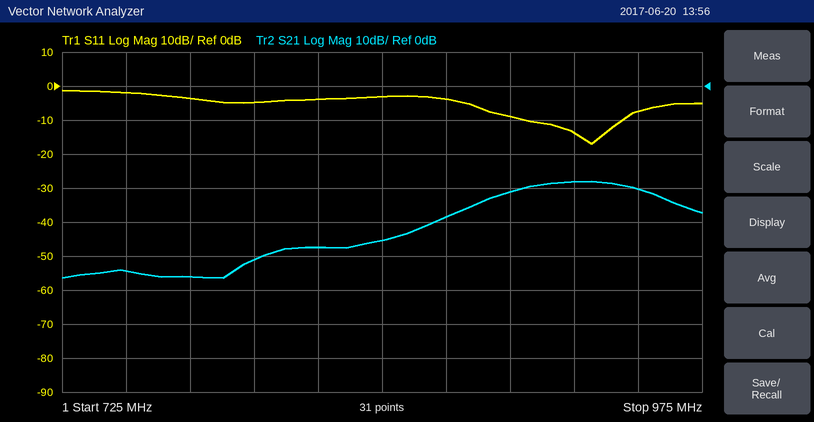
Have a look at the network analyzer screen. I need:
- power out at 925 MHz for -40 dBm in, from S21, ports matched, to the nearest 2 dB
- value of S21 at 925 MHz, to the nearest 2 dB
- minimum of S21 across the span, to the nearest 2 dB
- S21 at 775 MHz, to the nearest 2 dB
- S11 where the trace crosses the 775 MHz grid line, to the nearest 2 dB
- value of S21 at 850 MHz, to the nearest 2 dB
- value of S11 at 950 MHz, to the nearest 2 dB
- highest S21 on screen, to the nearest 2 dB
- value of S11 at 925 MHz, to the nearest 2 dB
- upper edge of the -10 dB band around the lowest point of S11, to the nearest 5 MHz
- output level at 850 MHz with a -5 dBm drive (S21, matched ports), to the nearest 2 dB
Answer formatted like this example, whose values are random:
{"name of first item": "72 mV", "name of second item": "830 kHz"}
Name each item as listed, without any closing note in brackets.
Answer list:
{"power out at 925 MHz for -40 dBm in, from S21, ports matched, to the nearest 2 dB": "-68 dBm", "value of S21 at 925 MHz, to the nearest 2 dB": "-28 dB", "minimum of S21 across the span, to the nearest 2 dB": "-56 dB", "S21 at 775 MHz, to the nearest 2 dB": "-56 dB", "S11 where the trace crosses the 775 MHz grid line, to the nearest 2 dB": "-4 dB", "value of S21 at 850 MHz, to the nearest 2 dB": "-46 dB", "value of S11 at 950 MHz, to the nearest 2 dB": "-8 dB", "highest S21 on screen, to the nearest 2 dB": "-28 dB", "value of S11 at 925 MHz, to the nearest 2 dB": "-14 dB", "upper edge of the -10 dB band around the lowest point of S11, to the nearest 5 MHz": "945 MHz", "output level at 850 MHz with a -5 dBm drive (S21, matched ports), to the nearest 2 dB": "-50 dBm"}
